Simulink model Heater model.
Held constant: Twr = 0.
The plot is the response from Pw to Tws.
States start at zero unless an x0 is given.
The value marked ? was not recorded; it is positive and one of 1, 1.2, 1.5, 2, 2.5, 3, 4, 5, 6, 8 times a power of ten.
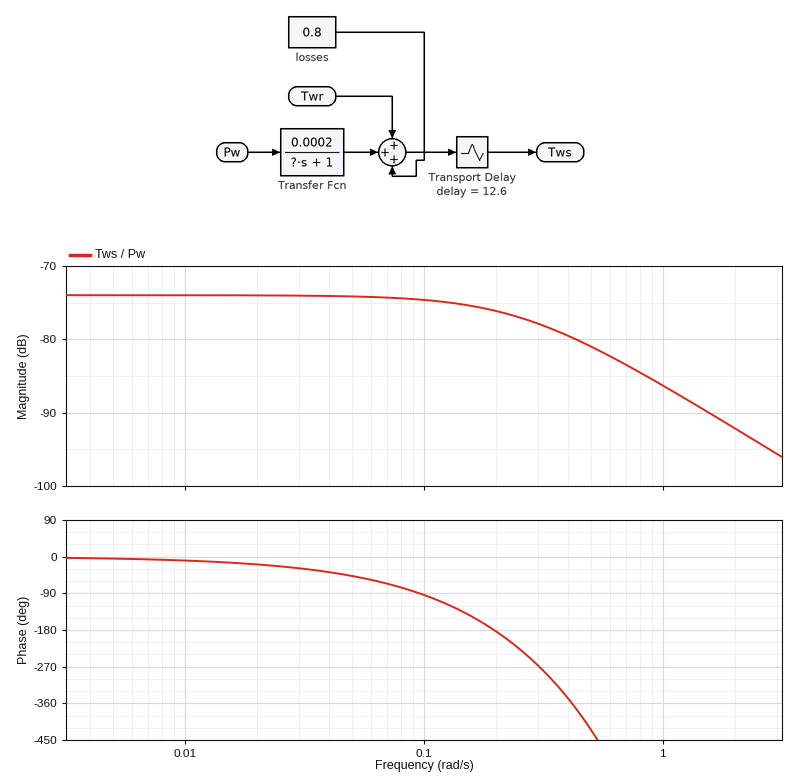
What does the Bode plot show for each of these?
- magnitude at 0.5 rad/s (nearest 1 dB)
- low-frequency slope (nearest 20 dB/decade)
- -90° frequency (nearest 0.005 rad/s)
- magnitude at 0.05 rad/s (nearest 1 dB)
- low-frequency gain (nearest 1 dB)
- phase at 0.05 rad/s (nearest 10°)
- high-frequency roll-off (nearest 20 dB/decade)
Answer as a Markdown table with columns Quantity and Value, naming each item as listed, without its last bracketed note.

| Quantity | Value |
|---|---|
| magnitude at 0.5 rad/s | -81 dB |
| low-frequency slope | 0 dB/decade |
| -90° frequency | 0.095 rad/s |
| magnitude at 0.05 rad/s | -74 dB |
| low-frequency gain | -74 dB |
| phase at 0.05 rad/s | -50° |
| high-frequency roll-off | -20 dB/decade |
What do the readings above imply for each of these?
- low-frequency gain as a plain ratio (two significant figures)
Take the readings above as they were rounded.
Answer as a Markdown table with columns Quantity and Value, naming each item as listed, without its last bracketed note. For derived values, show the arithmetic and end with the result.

| Quantity | Value |
|---|---|
| low-frequency gain as a plain ratio | 10^(-74 / 20) = 0.00020 |
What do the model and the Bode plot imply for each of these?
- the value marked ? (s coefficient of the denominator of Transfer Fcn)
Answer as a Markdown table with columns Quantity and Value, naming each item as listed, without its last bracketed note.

| Quantity | Value |
|---|---|
| the value marked ? | 4 |
